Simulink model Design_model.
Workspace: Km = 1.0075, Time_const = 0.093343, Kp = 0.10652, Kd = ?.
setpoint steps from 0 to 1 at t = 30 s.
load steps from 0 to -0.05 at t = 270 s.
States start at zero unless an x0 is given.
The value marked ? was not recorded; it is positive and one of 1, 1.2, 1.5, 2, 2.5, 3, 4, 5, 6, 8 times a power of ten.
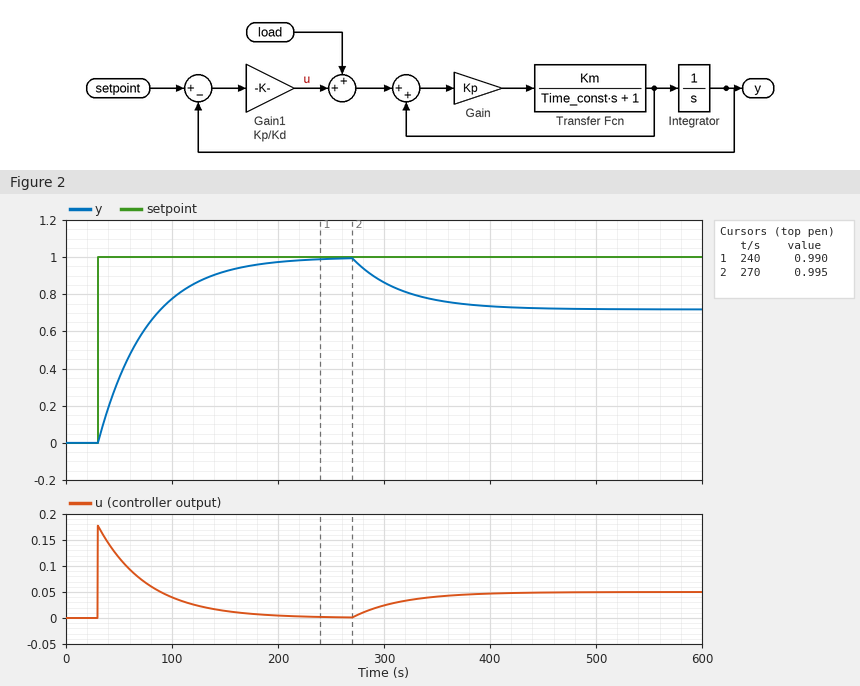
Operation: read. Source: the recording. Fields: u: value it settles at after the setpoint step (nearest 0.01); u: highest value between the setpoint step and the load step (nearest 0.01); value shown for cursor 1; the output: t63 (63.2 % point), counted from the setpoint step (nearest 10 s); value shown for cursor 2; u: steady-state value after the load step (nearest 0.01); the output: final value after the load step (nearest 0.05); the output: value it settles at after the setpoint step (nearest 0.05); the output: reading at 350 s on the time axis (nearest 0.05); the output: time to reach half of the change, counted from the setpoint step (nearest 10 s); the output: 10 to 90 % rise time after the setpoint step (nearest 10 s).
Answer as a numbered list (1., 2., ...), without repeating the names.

1. 0.00
2. 0.18
3. 0.990
4. 50 s
5. 0.995
6. 0.05
7. 0.70
8. 1.00
9. 0.75
10. 30 s
11. 100 s
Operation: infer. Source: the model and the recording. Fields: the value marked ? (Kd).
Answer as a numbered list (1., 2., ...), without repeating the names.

1. 0.6
